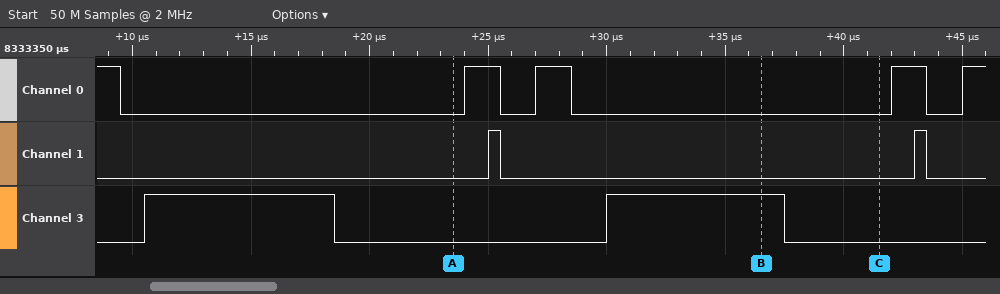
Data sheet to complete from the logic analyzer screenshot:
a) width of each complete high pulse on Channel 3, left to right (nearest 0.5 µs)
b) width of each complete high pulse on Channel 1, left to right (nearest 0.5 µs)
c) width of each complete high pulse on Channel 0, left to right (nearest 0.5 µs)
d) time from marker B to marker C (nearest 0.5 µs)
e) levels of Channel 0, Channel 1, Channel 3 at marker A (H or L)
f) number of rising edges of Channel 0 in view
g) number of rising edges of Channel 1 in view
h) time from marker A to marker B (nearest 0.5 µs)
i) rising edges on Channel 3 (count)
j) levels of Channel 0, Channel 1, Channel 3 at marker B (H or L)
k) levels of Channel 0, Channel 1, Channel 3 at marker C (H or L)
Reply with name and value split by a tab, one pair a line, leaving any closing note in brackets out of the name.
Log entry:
width of each complete high pulse on Channel 3, left to right	8 µs, 7.5 µs
width of each complete high pulse on Channel 1, left to right	0.5 µs, 0.5 µs
width of each complete high pulse on Channel 0, left to right	1.5 µs, 1.5 µs, 1.5 µs
time from marker B to marker C	5 µs
levels of Channel 0, Channel 1, Channel 3 at marker A	Channel 0=L, Channel 1=L, Channel 3=L
number of rising edges of Channel 0 in view	4
number of rising edges of Channel 1 in view	2
time from marker A to marker B	13 µs
rising edges on Channel 3	2
levels of Channel 0, Channel 1, Channel 3 at marker B	Channel 0=L, Channel 1=L, Channel 3=H
levels of Channel 0, Channel 1, Channel 3 at marker C	Channel 0=L, Channel 1=L, Channel 3=L
